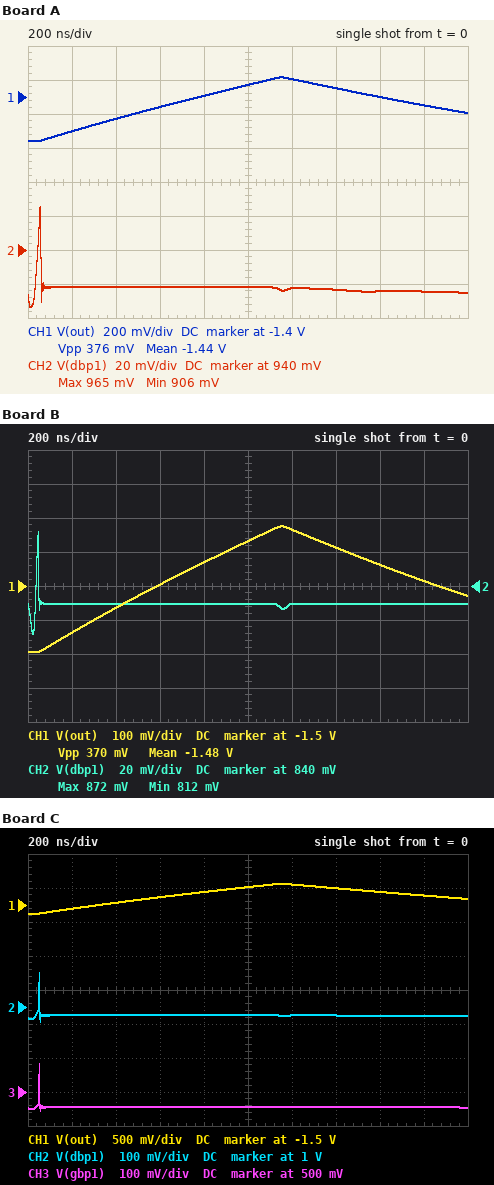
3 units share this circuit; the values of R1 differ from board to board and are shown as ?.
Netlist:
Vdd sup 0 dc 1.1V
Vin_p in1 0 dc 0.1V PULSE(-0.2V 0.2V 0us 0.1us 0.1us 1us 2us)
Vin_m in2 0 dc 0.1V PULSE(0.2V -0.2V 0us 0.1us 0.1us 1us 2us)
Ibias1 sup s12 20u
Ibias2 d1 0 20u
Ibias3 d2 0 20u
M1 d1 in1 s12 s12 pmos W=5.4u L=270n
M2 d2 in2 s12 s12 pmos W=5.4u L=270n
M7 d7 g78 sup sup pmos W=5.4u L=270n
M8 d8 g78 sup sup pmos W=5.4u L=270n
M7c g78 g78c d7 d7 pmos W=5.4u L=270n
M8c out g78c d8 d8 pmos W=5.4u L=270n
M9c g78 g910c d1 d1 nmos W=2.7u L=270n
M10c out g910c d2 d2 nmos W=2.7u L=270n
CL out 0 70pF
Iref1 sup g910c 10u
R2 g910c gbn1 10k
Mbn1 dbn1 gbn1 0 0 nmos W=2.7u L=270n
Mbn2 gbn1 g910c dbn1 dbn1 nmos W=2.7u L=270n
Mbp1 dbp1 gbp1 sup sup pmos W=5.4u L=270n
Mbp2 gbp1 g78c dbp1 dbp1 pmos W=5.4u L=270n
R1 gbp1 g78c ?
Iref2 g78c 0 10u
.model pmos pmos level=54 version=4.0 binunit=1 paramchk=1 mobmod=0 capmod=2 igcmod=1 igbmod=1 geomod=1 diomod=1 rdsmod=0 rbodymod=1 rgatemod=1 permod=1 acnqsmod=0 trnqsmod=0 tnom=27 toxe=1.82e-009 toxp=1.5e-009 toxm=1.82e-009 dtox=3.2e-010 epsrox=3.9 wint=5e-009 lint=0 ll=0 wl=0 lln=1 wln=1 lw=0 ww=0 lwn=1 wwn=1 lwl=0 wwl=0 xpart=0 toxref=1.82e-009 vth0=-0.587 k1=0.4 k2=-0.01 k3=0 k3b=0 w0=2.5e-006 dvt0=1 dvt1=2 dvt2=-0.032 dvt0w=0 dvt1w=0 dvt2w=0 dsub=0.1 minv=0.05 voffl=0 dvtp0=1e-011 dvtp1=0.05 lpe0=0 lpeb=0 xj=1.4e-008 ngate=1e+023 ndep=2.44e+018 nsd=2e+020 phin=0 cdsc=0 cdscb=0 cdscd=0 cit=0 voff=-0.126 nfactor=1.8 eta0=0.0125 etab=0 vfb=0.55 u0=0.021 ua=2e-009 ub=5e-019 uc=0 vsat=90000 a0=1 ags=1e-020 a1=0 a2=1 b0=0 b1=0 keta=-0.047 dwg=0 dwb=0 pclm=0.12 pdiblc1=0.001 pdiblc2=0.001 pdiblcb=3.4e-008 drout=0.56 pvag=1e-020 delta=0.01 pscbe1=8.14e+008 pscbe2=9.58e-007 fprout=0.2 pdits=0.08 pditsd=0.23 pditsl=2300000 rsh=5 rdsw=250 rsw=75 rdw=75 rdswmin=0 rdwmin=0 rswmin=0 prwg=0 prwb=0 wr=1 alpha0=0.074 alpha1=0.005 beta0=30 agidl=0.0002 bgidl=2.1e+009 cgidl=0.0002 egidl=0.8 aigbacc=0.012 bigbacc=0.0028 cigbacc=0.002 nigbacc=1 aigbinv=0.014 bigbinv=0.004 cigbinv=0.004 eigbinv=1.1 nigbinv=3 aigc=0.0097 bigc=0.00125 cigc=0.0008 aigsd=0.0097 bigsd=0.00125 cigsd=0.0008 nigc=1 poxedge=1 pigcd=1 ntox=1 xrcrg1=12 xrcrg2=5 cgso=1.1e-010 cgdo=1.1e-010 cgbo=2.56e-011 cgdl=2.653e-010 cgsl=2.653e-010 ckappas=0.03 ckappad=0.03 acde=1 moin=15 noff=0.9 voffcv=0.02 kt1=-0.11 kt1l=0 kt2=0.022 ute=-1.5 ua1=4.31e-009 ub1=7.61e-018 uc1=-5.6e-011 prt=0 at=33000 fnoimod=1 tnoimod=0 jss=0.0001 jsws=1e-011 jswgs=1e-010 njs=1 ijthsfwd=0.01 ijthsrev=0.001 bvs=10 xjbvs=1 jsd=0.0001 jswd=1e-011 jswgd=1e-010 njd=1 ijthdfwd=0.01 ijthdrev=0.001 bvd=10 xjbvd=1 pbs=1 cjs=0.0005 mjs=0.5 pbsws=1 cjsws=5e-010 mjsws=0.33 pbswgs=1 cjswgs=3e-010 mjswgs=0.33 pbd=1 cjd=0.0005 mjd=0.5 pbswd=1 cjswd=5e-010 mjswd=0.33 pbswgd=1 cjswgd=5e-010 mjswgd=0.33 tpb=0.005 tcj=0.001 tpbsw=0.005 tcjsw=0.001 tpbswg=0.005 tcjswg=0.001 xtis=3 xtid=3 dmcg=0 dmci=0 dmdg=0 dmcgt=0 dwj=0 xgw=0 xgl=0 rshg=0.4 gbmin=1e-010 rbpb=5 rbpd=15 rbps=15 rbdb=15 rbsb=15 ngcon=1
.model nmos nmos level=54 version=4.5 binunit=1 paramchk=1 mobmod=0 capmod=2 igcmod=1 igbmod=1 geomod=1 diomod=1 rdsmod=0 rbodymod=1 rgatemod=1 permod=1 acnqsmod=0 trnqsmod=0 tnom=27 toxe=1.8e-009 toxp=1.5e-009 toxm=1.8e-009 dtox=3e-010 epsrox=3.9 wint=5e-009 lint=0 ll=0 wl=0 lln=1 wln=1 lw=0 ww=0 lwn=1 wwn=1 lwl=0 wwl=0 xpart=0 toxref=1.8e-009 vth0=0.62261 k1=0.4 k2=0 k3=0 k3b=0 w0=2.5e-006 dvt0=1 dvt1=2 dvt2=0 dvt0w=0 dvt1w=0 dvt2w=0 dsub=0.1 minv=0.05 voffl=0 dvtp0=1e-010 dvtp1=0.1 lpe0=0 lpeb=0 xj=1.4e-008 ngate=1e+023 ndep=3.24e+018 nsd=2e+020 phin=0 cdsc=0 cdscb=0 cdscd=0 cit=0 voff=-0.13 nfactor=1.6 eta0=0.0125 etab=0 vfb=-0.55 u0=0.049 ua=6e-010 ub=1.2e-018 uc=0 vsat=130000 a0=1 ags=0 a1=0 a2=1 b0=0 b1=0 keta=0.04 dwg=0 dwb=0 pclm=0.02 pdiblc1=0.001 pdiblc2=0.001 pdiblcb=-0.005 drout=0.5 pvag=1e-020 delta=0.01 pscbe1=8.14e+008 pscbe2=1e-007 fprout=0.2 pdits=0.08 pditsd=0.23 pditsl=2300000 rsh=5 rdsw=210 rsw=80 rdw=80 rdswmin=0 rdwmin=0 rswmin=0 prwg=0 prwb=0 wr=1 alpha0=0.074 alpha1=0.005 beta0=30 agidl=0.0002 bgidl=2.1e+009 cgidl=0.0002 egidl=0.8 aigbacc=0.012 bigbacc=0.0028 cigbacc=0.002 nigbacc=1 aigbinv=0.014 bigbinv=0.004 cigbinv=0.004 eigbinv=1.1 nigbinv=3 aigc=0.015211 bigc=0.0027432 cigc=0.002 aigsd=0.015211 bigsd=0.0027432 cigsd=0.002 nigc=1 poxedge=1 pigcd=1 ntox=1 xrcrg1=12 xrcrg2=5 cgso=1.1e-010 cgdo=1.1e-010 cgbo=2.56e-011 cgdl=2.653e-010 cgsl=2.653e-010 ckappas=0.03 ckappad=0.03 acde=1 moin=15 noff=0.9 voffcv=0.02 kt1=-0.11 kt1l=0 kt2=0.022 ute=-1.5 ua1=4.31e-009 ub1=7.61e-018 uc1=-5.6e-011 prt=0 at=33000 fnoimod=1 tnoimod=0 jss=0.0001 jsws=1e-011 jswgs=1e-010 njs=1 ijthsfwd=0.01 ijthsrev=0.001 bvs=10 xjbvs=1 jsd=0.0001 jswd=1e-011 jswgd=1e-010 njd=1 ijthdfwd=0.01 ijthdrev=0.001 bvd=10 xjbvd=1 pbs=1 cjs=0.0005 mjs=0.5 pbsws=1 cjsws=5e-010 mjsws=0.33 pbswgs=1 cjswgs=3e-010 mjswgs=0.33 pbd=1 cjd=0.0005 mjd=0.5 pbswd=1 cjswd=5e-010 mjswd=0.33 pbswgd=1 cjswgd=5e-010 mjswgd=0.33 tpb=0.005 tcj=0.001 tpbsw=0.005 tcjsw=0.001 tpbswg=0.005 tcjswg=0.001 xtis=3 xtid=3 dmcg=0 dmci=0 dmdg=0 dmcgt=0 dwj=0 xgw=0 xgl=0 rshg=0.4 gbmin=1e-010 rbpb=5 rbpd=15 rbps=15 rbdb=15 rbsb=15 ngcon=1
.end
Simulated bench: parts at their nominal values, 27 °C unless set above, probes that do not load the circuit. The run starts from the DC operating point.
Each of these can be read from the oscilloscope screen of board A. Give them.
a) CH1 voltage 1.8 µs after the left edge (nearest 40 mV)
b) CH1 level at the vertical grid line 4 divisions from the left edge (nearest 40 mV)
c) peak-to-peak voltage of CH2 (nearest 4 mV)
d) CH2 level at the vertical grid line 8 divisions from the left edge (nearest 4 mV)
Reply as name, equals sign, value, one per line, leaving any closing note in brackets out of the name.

CH1 voltage 1.8 µs after the left edge = -1.44 V
CH1 level at the vertical grid line 4 divisions from the left edge = -1.40 V
peak-to-peak voltage of CH2 = 60 mV
CH2 level at the vertical grid line 8 divisions from the left edge = 916 mV
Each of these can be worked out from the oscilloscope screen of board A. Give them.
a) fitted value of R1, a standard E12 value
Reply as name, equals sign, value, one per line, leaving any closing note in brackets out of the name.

fitted value of R1, a standard E12 value = 18 kΩ
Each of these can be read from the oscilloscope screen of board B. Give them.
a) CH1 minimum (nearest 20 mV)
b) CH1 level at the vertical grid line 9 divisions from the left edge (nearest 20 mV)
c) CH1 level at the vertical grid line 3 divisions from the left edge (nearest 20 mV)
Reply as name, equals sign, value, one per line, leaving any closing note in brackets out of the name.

CH1 minimum = -1.70 V
CH1 level at the vertical grid line 9 divisions from the left edge = -1.48 V
CH1 level at the vertical grid line 3 divisions from the left edge = -1.50 V
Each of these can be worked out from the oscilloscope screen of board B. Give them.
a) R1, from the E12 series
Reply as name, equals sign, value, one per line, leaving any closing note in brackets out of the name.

R1, from the E12 series = 27 kΩ
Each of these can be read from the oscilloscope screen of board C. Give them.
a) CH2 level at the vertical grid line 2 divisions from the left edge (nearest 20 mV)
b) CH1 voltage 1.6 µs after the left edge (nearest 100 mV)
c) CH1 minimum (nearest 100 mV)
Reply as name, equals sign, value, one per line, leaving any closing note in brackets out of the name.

CH2 level at the vertical grid line 2 divisions from the left edge = 980 mV
CH1 voltage 1.6 µs after the left edge = -1.3 V
CH1 minimum = -1.6 V
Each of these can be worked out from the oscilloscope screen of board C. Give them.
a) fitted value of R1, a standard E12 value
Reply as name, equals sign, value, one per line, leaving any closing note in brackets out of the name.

fitted value of R1, a standard E12 value = 12 kΩ
